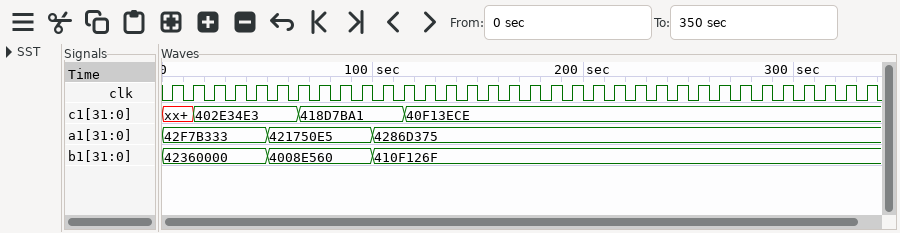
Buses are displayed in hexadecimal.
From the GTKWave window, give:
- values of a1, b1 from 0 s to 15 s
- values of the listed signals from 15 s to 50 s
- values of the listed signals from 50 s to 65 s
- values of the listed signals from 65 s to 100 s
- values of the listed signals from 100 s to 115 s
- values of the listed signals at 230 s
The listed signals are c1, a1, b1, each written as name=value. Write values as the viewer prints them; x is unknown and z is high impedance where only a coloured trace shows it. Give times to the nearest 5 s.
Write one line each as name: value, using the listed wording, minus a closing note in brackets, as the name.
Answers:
values of a1, b1 from 0 s to 15 s: a1=42F7B333, b1=42360000
values of the listed signals from 15 s to 50 s: c1=402E34E3, a1=42F7B333, b1=42360000
values of the listed signals from 50 s to 65 s: c1=402E34E3, a1=421750E5, b1=4008E560
values of the listed signals from 65 s to 100 s: c1=418D7BA1, a1=421750E5, b1=4008E560
values of the listed signals from 100 s to 115 s: c1=418D7BA1, a1=4286D375, b1=410F126F
values of the listed signals at 230 s: c1=40F13ECE, a1=4286D375, b1=410F126F
